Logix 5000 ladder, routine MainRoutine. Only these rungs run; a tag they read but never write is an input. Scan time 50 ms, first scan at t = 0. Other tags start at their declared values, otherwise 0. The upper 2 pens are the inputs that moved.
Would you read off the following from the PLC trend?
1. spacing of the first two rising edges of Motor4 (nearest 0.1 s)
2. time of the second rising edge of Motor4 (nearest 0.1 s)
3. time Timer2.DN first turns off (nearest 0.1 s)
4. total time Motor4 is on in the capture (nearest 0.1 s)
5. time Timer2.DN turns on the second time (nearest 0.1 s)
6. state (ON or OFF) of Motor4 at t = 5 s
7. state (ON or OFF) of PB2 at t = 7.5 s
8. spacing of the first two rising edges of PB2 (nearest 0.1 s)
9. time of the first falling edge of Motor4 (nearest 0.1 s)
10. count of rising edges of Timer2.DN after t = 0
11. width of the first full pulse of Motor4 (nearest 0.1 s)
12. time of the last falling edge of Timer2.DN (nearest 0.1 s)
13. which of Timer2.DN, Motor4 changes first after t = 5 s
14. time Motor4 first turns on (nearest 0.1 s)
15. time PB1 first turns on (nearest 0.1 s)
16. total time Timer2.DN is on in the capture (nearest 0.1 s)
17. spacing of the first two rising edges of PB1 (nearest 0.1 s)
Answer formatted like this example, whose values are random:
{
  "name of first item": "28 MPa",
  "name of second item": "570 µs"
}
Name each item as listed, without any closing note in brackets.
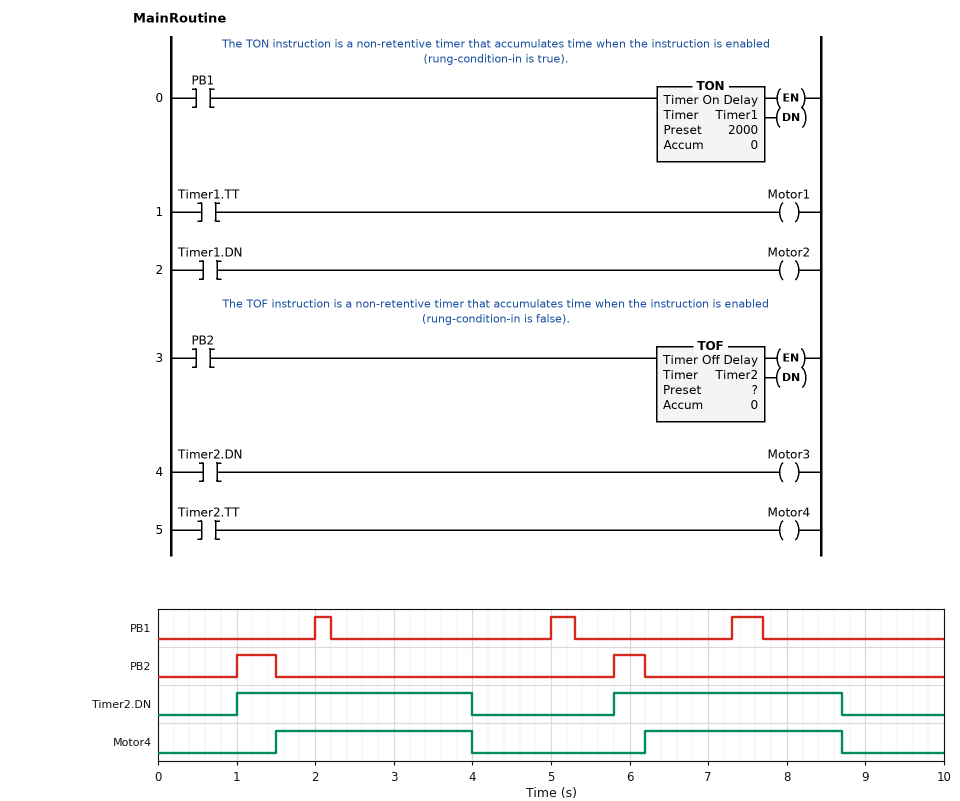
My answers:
{
  "spacing of the first two rising edges of Motor4": "4.7 s",
  "time of the second rising edge of Motor4": "6.2 s",
  "time Timer2.DN first turns off": "4.0 s",
  "total time Motor4 is on in the capture": "5.0 s",
  "time Timer2.DN turns on the second time": "5.8 s",
  "state (ON or OFF) of Motor4 at t = 5 s": "OFF",
  "state (ON or OFF) of PB2 at t = 7.5 s": "OFF",
  "spacing of the first two rising edges of PB2": "4.8 s",
  "time of the first falling edge of Motor4": "4.0 s",
  "count of rising edges of Timer2.DN after t = 0": "2",
  "width of the first full pulse of Motor4": "2.5 s",
  "time of the last falling edge of Timer2.DN": "8.7 s",
  "which of Timer2.DN, Motor4 changes first after t = 5 s": "Timer2.DN",
  "time Motor4 first turns on": "1.5 s",
  "time PB1 first turns on": "2.0 s",
  "total time Timer2.DN is on in the capture": "5.9 s",
  "spacing of the first two rising edges of PB1": "3.0 s"
}
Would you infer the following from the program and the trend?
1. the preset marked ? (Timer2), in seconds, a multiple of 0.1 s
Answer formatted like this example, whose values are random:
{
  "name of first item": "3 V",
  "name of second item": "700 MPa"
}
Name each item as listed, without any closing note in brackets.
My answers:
{
  "the preset marked ? (Timer2), in seconds, a multiple of 0.1 s": "2.5 s"
}
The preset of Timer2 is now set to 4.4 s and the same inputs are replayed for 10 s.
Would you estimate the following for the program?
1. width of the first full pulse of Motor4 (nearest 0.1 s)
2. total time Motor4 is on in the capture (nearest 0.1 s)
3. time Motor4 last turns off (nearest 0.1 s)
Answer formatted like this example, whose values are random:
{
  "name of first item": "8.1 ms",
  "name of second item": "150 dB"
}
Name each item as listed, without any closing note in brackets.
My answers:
{
  "width of the first full pulse of Motor4": "4.3 s",
  "total time Motor4 is on in the capture": "8.1 s",
  "time Motor4 last turns off": "5.8 s"
}
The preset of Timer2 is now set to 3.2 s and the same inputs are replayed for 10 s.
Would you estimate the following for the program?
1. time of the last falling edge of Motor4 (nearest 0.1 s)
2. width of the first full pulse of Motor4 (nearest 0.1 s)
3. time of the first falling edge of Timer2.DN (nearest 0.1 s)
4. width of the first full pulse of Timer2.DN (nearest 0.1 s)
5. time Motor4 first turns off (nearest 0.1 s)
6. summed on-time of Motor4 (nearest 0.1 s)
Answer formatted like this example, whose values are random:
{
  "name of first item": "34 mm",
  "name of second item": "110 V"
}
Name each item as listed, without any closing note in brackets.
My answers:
{
  "time of the last falling edge of Motor4": "9.4 s",
  "width of the first full pulse of Motor4": "3.2 s",
  "time of the first falling edge of Timer2.DN": "4.7 s",
  "width of the first full pulse of Timer2.DN": "3.7 s",
  "time Motor4 first turns off": "4.7 s",
  "summed on-time of Motor4": "6.4 s"
}
